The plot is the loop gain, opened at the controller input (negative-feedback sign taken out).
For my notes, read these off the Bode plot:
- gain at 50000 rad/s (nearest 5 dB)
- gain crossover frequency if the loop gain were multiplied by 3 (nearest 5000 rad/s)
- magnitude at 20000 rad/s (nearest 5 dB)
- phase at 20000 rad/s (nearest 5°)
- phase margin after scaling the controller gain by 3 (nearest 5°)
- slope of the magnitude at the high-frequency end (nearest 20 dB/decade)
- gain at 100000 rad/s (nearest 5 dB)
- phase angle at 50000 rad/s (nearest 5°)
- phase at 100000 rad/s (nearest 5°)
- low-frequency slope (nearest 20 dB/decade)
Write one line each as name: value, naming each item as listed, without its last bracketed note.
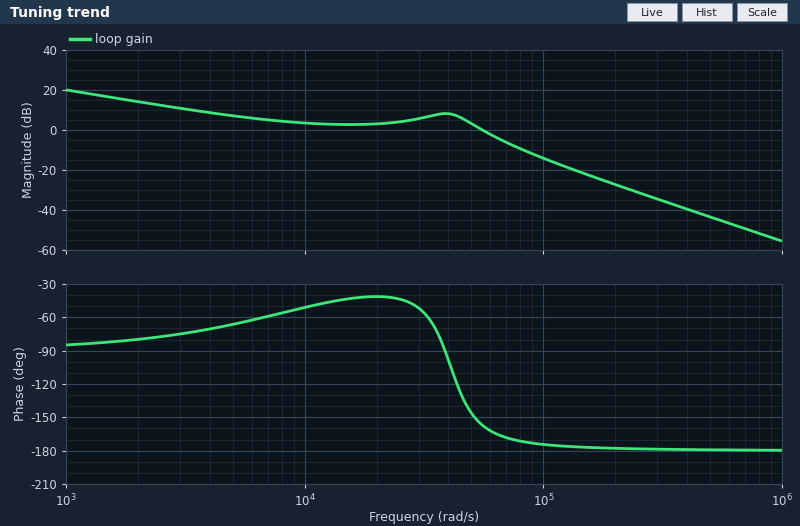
gain at 50000 rad/s: 5 dB
gain crossover frequency if the loop gain were multiplied by 3: 80000 rad/s
magnitude at 20000 rad/s: 5 dB
phase at 20000 rad/s: -40°
phase margin after scaling the controller gain by 3: 10°
slope of the magnitude at the high-frequency end: -40 dB/decade
gain at 100000 rad/s: -15 dB
phase angle at 50000 rad/s: -145°
phase at 100000 rad/s: -175°
low-frequency slope: -20 dB/decade
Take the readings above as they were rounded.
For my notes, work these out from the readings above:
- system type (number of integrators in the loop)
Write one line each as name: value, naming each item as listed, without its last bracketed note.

system type: 1
